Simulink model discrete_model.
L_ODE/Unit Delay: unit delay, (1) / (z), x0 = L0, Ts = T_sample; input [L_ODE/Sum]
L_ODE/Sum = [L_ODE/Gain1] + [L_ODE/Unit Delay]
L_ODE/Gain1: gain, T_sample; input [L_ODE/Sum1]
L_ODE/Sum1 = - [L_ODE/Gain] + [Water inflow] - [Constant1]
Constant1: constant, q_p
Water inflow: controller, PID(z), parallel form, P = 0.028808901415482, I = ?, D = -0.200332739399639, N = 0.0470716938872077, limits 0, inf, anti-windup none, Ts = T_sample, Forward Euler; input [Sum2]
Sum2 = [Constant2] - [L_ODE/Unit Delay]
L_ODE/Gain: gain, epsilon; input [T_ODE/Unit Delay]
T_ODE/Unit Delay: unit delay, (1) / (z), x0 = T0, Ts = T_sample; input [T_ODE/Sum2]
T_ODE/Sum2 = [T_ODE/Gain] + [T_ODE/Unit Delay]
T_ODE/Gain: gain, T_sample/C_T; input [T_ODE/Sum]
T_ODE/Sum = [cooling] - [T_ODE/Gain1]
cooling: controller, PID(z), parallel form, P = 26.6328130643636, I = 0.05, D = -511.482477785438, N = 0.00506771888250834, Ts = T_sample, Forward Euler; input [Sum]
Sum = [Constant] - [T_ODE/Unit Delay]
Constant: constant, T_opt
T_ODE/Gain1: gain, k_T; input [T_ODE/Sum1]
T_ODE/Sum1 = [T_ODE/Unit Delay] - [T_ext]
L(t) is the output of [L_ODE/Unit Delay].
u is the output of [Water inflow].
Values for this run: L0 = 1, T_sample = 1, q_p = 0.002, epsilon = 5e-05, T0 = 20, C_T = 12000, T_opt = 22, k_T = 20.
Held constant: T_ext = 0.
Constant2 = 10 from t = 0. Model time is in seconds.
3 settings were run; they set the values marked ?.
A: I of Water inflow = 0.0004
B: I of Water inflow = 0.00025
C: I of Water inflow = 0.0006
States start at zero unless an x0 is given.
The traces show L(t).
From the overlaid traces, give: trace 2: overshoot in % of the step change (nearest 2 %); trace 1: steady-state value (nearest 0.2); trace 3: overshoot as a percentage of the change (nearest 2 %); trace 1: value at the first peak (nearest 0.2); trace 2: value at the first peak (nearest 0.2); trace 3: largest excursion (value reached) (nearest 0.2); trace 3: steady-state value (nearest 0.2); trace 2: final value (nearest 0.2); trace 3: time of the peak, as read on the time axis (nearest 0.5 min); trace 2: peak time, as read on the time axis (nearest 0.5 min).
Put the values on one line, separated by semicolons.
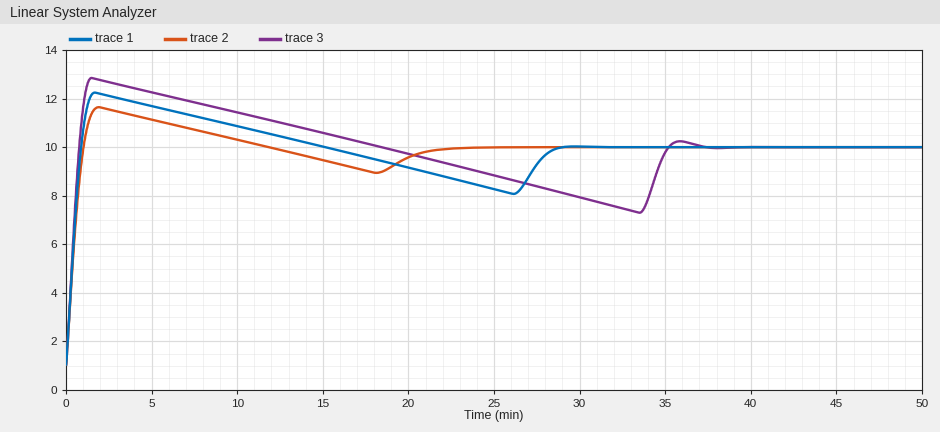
18 %; 10.0; 32 %; 12.2; 11.6; 12.8; 10.0; 10.0; 1.5 min; 2.0 min
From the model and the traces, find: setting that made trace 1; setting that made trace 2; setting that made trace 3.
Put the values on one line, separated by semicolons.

A; B; C
